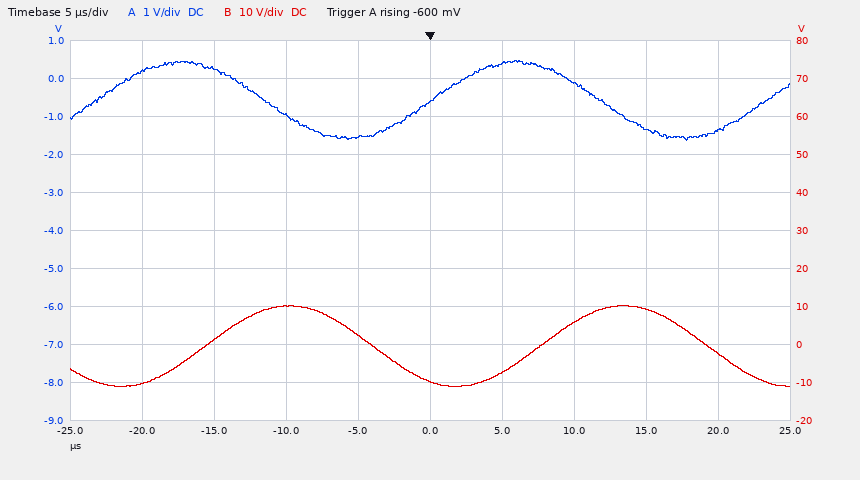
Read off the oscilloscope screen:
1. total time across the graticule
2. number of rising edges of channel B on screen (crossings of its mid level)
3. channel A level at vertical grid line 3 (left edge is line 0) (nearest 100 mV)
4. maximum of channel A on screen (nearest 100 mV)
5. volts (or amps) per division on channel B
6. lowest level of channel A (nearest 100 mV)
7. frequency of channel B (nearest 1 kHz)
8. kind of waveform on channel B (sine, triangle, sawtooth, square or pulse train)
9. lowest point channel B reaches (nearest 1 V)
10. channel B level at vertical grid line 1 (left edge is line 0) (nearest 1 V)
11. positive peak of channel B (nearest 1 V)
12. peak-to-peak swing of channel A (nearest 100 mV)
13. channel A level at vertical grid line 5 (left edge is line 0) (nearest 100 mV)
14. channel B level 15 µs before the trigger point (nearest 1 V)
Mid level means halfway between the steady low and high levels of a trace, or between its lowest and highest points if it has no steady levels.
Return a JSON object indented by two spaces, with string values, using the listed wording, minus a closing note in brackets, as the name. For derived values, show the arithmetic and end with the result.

{
  "total time across the graticule": "50 µs",
  "number of rising edges of channel B on screen": "2",
  "channel A level at vertical grid line 3 (left edge is line 0)": "-1.0 V",
  "maximum of channel A on screen": "500 mV",
  "volts (or amps) per division on channel B": "10 V",
  "lowest level of channel A": "-1.6 V",
  "frequency of channel B": "43 kHz",
  "kind of waveform on channel B": "sine",
  "lowest point channel B reaches": "-11 V",
  "channel B level at vertical grid line 1 (left edge is line 0)": "-10 V",
  "positive peak of channel B": "10 V",
  "peak-to-peak swing of channel A": "500 mV − (-1.6 V) = 2.1 V",
  "channel A level at vertical grid line 5 (left edge is line 0)": "-600 mV",
  "channel B level 15 µs before the trigger point": "1 V"
}
